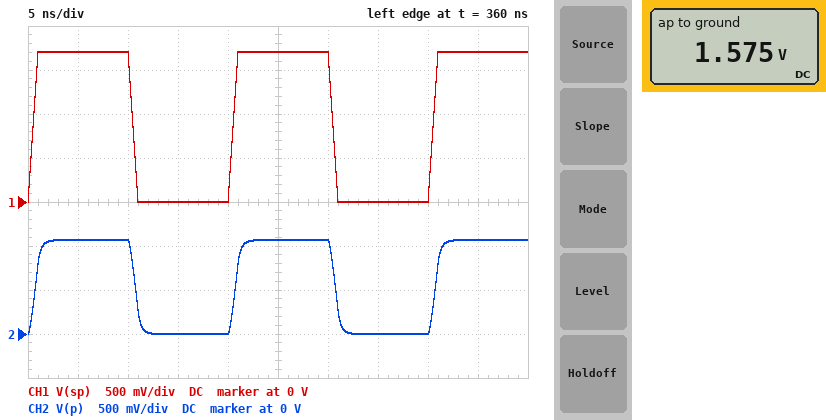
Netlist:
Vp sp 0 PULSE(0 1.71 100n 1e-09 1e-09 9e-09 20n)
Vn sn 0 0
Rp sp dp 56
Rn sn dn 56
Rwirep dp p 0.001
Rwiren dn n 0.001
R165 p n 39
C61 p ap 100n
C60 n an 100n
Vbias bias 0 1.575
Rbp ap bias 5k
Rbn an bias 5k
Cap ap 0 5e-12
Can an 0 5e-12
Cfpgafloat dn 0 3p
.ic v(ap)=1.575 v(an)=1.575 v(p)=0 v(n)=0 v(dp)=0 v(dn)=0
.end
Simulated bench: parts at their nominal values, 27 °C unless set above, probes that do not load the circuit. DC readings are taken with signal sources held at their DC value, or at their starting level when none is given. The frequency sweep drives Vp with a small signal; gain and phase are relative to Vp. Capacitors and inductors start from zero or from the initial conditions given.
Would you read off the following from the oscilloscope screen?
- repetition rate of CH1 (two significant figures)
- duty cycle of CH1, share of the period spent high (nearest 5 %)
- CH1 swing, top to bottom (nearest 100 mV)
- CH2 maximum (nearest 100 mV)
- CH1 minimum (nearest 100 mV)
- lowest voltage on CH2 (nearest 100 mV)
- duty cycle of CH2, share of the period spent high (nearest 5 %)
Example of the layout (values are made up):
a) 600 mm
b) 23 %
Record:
a) 50 MHz
b) 50 %
c) 1.7 V
d) 1.1 V
e) 0 V
f) 0 V
g) 50 %
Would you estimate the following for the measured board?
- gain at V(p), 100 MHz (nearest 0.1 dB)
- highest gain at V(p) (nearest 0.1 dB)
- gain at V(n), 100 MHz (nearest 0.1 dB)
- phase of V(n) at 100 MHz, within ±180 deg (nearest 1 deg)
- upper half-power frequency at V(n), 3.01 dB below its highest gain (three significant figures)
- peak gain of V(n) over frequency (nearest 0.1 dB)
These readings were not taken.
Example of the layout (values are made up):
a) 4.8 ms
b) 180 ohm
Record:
a) -4.3 dB
b) -4.1 dB
c) -9.0 dB
d) -16 deg
e) 413 MHz
f) -8.7 dB
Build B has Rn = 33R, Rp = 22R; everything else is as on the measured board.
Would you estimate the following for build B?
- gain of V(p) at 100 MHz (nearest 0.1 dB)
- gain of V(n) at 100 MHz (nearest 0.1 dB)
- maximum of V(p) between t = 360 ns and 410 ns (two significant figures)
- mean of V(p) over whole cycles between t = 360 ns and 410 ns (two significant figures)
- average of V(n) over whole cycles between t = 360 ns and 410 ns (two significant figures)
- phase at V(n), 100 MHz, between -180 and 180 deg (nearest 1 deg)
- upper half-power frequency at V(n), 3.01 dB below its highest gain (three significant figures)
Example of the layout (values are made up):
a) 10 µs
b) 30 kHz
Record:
a) -2.4 dB
b) -9.2 dB
c) 1.3 V
d) 650 mV
e) 300 mV
f) -9 deg
g) 758 MHz
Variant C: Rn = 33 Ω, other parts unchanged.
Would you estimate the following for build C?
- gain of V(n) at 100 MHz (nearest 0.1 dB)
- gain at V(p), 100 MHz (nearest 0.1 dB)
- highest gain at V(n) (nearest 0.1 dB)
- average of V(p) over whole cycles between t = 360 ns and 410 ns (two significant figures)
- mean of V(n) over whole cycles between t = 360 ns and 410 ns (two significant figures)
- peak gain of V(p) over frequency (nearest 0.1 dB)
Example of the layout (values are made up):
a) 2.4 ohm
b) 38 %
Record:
a) -12.0 dB
b) -5.2 dB
c) -11.9 dB
d) 480 mV
e) 220 mV
f) -5.1 dB
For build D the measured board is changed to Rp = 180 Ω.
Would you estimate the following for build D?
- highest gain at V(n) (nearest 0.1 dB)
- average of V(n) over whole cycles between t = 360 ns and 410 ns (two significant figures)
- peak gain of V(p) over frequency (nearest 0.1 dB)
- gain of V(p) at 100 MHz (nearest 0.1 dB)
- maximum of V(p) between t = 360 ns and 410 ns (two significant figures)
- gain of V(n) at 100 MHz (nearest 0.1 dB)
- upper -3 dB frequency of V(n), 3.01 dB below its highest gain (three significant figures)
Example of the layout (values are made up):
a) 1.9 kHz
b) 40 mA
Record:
a) -14.0 dB
b) 170 mV
c) -9.4 dB
d) -9.8 dB
e) 580 mV
f) -14.5 dB
g) 277 MHz
